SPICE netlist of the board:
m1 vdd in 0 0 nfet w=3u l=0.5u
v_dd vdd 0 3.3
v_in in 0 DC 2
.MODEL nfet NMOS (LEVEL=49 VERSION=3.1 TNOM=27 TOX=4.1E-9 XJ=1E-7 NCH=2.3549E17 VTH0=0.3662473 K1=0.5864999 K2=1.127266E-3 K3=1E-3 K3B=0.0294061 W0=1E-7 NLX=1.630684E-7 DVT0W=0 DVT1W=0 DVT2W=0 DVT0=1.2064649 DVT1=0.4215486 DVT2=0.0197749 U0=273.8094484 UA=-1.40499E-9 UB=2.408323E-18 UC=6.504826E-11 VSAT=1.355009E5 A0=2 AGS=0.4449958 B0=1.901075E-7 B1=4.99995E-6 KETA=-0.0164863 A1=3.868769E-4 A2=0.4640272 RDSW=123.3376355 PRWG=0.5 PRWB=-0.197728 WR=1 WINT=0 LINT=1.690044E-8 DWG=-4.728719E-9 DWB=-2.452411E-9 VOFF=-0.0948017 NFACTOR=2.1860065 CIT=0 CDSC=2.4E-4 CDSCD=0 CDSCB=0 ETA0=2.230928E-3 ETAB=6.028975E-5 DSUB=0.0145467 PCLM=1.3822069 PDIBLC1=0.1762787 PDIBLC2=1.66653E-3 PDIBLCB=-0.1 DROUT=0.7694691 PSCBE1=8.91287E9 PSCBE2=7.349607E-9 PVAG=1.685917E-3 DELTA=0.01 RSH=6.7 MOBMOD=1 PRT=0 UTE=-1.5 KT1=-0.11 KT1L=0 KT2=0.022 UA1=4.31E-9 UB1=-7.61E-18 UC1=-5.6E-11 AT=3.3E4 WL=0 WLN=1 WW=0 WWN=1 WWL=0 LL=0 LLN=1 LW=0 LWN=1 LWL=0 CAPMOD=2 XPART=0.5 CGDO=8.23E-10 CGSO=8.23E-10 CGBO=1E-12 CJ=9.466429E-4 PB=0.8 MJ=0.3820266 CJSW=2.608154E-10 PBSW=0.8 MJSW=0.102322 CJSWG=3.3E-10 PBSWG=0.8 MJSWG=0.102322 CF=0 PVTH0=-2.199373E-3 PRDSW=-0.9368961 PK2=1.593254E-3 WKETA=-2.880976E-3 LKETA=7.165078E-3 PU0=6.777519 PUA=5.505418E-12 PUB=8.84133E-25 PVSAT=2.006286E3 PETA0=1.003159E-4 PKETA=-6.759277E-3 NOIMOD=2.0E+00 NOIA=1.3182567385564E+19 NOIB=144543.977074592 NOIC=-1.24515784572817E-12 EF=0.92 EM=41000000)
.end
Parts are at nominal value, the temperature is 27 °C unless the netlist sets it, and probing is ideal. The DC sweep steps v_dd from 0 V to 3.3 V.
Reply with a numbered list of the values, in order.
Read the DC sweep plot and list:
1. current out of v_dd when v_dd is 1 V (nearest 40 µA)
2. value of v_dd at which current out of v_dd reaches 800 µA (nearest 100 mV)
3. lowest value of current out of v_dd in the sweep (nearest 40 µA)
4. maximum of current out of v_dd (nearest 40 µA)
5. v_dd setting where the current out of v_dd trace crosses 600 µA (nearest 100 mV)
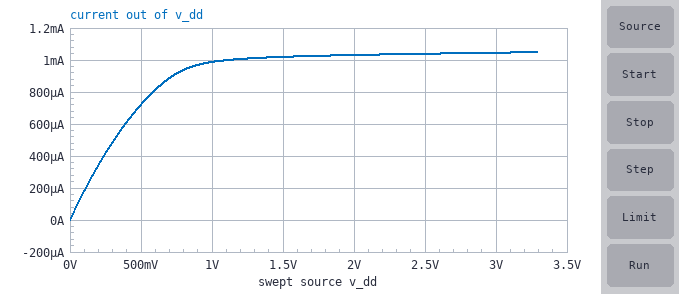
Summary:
1. 1.00 mA
2. 600 mV
3. 0 A
4. 1.04 mA
5. 400 mV
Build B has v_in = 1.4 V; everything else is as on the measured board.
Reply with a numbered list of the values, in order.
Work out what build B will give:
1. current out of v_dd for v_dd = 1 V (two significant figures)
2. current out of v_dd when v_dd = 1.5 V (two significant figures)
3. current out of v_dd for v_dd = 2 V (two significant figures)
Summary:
1. 500 µA
2. 510 µA
3. 520 µA
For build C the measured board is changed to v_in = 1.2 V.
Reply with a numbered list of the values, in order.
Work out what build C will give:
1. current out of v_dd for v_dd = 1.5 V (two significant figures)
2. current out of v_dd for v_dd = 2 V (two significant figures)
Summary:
1. 350 µA
2. 360 µA
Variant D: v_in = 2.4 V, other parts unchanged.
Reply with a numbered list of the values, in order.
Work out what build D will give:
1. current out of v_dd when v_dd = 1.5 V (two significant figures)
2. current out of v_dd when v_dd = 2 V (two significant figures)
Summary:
1. 1.3 mA
2. 1.4 mA
